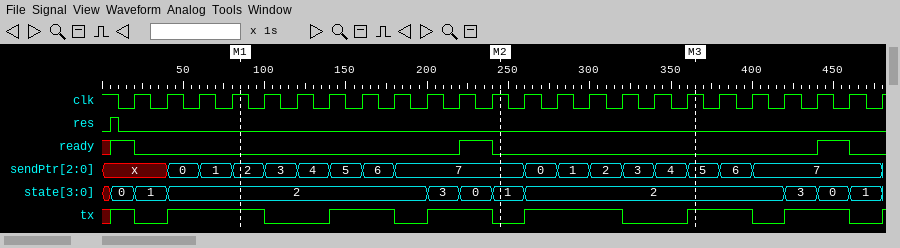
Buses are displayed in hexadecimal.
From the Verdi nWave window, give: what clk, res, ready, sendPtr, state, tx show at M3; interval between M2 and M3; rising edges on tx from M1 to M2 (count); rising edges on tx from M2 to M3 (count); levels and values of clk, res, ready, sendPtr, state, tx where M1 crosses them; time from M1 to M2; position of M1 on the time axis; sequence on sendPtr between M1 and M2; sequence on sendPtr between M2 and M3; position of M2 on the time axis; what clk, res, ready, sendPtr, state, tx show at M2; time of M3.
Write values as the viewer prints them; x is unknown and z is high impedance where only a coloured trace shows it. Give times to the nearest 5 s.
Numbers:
clk=1, res=0, ready=0, sendPtr=5, state=2, tx=1
120 s
2
2
clk=1, res=0, ready=0, sendPtr=2, state=2, tx=1
160 s
85 s
2, 3, 4, 5, 6, 7
7, 0, 1, 2, 3, 4, 5
245 s
clk=1, res=0, ready=0, sendPtr=7, state=1, tx=0
365 s
